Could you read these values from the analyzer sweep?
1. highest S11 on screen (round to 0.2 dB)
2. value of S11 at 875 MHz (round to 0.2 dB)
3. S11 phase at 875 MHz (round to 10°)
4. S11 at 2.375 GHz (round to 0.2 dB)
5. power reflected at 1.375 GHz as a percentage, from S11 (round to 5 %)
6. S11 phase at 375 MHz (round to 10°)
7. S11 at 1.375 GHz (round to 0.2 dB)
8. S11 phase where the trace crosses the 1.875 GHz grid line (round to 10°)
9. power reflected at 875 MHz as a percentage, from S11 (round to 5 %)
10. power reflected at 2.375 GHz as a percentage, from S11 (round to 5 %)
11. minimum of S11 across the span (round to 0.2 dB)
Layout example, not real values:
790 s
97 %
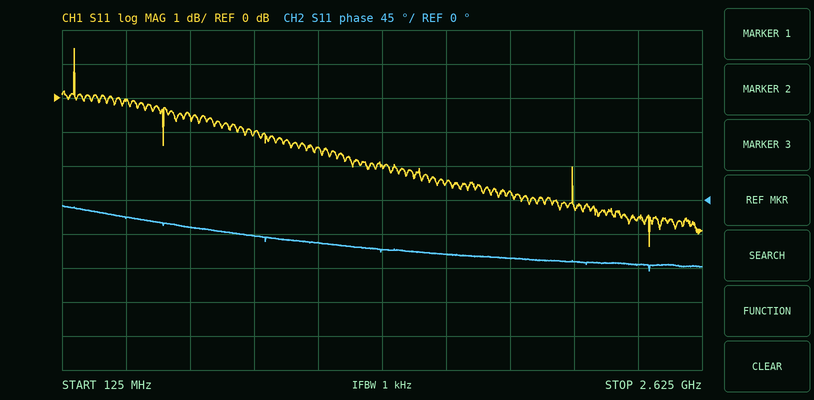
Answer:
1.4 dB
-1.0 dB
-50°
-3.6 dB
65 %
-20°
-2.0 dB
-80°
80 %
45 %
-4.4 dB
